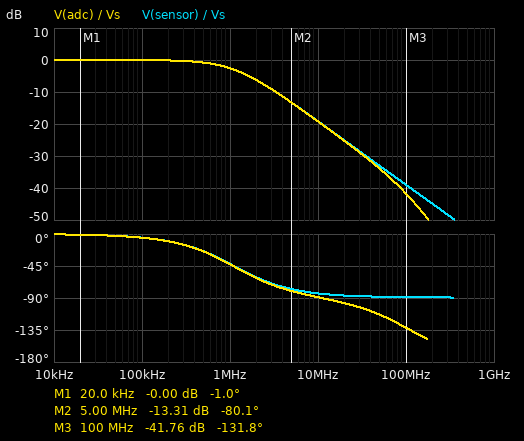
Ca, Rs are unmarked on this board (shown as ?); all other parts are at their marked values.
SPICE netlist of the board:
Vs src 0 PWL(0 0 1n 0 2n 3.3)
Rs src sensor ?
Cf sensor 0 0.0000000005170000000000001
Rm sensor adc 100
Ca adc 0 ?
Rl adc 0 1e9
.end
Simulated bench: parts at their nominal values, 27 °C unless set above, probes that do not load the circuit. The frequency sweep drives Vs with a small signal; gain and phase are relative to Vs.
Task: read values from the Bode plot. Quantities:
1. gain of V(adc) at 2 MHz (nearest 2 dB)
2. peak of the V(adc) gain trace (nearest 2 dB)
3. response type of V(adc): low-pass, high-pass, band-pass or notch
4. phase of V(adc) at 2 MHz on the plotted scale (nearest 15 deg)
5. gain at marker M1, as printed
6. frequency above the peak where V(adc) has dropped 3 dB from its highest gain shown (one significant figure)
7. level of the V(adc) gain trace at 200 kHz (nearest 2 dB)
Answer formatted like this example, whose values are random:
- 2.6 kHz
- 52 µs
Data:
- -6 dB
- 0 dB
- low-pass
- -60 deg
- -0.00 dB
- 1 MHz
- 0 dB
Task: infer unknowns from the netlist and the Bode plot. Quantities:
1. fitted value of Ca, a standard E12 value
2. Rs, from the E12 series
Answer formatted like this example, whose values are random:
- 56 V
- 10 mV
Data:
- 15 pF
- 270 Ω
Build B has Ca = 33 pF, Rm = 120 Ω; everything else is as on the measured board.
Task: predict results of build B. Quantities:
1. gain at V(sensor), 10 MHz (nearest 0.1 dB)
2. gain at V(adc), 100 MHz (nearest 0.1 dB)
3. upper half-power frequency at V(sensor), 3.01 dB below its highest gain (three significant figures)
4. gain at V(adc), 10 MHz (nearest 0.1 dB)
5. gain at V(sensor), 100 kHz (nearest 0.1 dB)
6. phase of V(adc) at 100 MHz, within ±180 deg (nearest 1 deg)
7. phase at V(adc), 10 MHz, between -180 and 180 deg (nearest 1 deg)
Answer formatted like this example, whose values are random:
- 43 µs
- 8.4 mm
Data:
- -19.4 dB
- -47.5 dB
- 1.07 MHz
- -19.7 dB
- 0 dB
- -156 deg
- -97 deg
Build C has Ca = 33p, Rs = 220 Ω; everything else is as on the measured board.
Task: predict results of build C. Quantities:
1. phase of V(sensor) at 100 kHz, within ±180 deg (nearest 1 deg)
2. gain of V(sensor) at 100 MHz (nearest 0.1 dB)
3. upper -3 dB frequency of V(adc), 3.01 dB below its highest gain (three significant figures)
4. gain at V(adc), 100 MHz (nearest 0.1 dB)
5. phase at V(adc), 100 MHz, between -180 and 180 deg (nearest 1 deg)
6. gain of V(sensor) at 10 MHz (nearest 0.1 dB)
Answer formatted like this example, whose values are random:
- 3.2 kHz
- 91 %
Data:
- -4 deg
- -37.2 dB
- 1.31 MHz
- -44.4 dB
- -152 deg
- -17.7 dB
